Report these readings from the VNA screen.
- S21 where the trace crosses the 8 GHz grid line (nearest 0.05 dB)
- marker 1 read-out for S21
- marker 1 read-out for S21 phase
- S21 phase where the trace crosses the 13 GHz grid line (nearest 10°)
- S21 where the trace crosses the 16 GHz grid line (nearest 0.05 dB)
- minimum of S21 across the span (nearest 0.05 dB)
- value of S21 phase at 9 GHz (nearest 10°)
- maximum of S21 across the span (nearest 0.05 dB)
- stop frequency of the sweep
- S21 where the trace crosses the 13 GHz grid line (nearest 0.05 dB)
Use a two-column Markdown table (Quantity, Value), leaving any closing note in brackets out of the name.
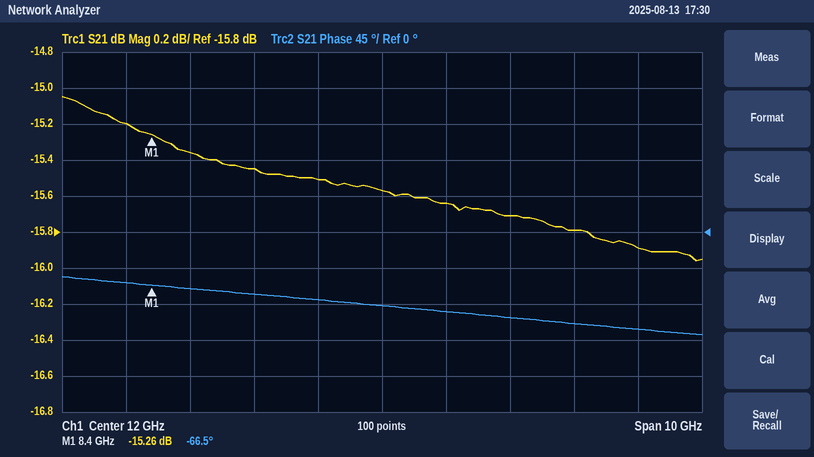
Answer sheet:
| Quantity | Value |
|---|---|
| S21 where the trace crosses the 8 GHz grid line | -15.20 dB |
| marker 1 read-out for S21 | -15.26 dB |
| marker 1 read-out for S21 phase | -66.5° |
| S21 phase where the trace crosses the 13 GHz grid line | -100° |
| S21 where the trace crosses the 16 GHz grid line | -15.90 dB |
| minimum of S21 across the span | -15.95 dB |
| value of S21 phase at 9 GHz | -70° |
| maximum of S21 across the span | -15.05 dB |
| stop frequency of the sweep | 17 GHz |
| S21 where the trace crosses the 13 GHz grid line | -15.65 dB |
